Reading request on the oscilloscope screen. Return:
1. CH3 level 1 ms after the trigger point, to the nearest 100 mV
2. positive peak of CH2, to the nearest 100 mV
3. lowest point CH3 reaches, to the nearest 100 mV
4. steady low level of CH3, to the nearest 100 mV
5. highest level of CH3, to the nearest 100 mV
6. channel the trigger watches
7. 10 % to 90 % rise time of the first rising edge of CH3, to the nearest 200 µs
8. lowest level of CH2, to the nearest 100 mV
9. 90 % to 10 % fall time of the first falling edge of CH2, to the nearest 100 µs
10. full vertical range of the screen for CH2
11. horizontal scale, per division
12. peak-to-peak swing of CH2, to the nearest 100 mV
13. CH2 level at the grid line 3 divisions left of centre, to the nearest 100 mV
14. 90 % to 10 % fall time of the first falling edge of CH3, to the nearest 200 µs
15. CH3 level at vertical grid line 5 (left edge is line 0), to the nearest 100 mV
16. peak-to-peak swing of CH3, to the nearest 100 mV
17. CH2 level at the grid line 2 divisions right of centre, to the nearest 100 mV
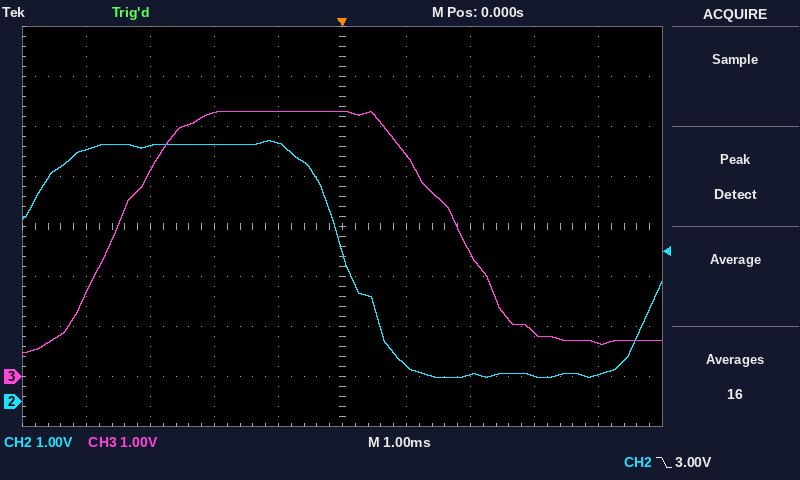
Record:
4.4 V
5.2 V
500 mV
700 mV
5.3 V
CH2
1.6 ms
500 mV
1.3 ms
8 V
1 ms
4.7 V
5.1 V
1.8 ms
5.3 V
4.8 V
500 mV
